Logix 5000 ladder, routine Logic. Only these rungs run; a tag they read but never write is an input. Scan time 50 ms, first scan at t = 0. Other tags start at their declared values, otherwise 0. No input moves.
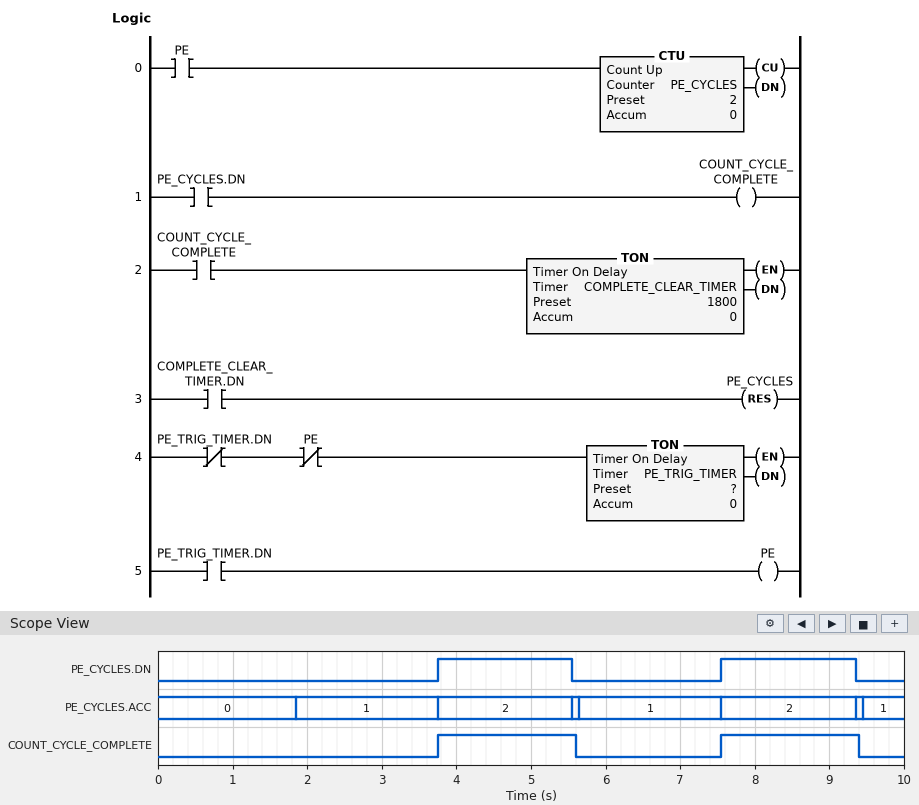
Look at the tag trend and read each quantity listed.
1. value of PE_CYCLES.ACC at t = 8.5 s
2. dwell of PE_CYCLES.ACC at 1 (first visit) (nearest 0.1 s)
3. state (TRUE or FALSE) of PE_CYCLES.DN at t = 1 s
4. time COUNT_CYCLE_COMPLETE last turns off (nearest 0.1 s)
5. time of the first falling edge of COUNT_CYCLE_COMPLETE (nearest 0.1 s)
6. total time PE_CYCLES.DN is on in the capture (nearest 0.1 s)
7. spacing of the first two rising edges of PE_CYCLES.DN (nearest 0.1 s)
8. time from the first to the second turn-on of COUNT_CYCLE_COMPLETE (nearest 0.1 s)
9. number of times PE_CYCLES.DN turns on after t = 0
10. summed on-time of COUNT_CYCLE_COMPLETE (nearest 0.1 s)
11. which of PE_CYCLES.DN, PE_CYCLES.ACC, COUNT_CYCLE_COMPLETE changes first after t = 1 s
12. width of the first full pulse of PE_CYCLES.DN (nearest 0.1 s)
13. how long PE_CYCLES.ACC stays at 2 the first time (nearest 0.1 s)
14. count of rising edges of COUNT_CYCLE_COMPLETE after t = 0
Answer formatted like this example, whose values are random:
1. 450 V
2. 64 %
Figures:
1. 2
2. 1.9 s
3. FALSE
4. 9.4 s
5. 5.6 s
6. 3.6 s
7. 3.8 s
8. 3.8 s
9. 2
10. 3.7 s
11. PE_CYCLES.ACC
12. 1.8 s
13. 1.8 s
14. 2
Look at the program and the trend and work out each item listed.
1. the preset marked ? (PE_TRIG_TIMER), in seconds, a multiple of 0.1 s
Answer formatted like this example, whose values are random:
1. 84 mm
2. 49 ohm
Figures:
1. 1.8 s
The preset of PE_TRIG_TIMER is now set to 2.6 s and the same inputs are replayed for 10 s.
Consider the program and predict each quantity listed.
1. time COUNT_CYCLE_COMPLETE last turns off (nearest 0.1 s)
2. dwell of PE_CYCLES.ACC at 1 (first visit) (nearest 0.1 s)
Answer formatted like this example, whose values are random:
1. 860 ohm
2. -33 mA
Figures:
1. 7.2 s
2. 2.7 s
